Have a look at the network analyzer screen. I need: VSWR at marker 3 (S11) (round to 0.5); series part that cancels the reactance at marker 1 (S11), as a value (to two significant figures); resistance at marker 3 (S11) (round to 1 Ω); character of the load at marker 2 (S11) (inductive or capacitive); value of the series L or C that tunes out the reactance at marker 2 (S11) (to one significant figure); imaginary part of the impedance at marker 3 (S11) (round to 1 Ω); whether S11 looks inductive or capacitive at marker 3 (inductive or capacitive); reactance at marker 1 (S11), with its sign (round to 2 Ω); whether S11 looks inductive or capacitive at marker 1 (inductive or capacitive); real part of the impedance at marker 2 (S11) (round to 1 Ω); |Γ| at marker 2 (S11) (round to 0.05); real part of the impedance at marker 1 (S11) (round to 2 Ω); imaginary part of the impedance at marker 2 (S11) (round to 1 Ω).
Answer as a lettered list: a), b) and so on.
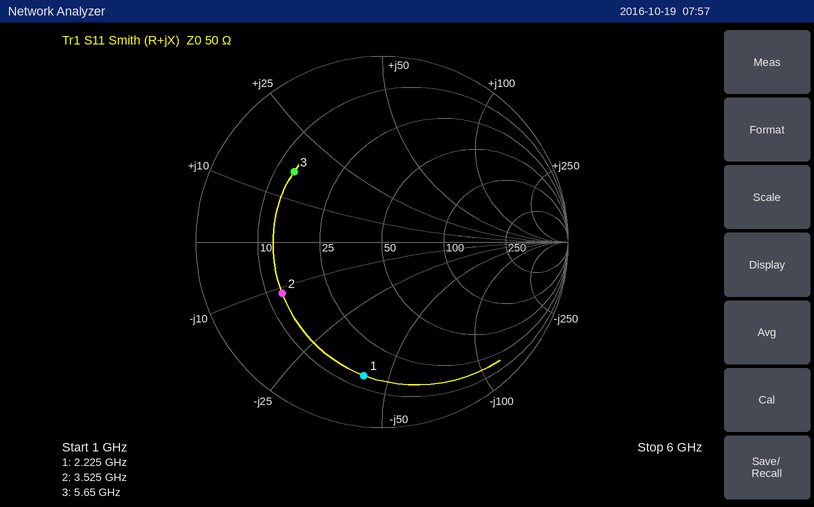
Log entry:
a) 4.0
b) 3.0 nH
c) 14 Ω
d) capacitive
e) 500 pH
f) +16 Ω
g) inductive
h) -42 Ω
i) capacitive
j) 13 Ω
k) 0.60
l) 14 Ω
m) -11 Ω
